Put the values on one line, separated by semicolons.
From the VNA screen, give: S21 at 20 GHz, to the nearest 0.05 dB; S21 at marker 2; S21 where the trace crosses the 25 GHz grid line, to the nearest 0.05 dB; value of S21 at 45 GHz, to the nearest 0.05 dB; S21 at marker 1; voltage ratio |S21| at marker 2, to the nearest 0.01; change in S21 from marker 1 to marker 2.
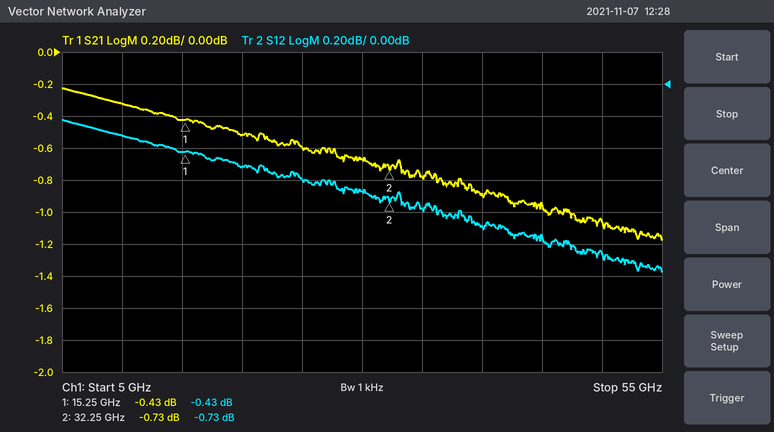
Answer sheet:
-0.50 dB; -0.73 dB; -0.60 dB; -0.95 dB; -0.43 dB; 0.92; -0.30 dB
